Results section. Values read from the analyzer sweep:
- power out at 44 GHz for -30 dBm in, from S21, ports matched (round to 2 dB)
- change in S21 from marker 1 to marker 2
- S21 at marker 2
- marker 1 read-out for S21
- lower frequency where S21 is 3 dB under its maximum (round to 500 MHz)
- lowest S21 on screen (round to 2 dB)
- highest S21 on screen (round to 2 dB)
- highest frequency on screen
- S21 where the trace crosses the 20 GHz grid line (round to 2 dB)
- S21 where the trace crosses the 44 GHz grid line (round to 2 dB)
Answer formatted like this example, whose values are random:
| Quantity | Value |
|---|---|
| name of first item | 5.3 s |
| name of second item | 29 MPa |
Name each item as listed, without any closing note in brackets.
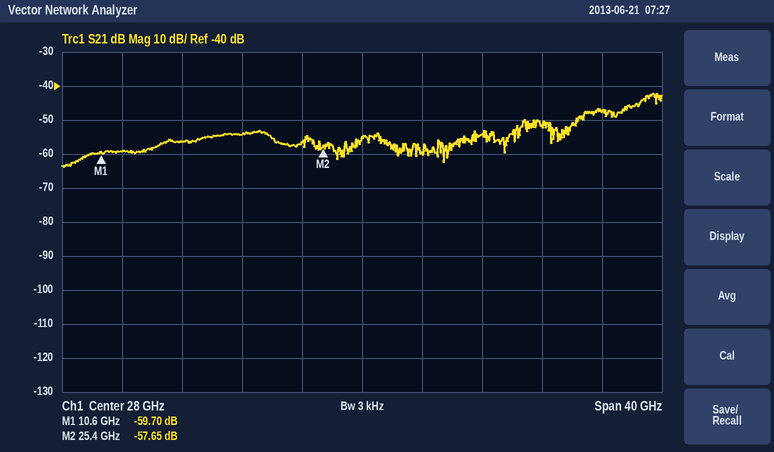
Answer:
| Quantity | Value |
|---|---|
| power out at 44 GHz for -30 dBm in, from S21, ports matched | -78 dBm |
| change in S21 from marker 1 to marker 2 | 2.05 dB |
| S21 at marker 2 | -57.65 dB |
| marker 1 read-out for S21 | -59.70 dB |
| lower frequency where S21 is 3 dB under its maximum | 46.5 GHz |
| lowest S21 on screen | -64 dB |
| highest S21 on screen | -42 dB |
| highest frequency on screen | 48 GHz |
| S21 where the trace crosses the 20 GHz grid line | -54 dB |
| S21 where the trace crosses the 44 GHz grid line | -48 dB |
